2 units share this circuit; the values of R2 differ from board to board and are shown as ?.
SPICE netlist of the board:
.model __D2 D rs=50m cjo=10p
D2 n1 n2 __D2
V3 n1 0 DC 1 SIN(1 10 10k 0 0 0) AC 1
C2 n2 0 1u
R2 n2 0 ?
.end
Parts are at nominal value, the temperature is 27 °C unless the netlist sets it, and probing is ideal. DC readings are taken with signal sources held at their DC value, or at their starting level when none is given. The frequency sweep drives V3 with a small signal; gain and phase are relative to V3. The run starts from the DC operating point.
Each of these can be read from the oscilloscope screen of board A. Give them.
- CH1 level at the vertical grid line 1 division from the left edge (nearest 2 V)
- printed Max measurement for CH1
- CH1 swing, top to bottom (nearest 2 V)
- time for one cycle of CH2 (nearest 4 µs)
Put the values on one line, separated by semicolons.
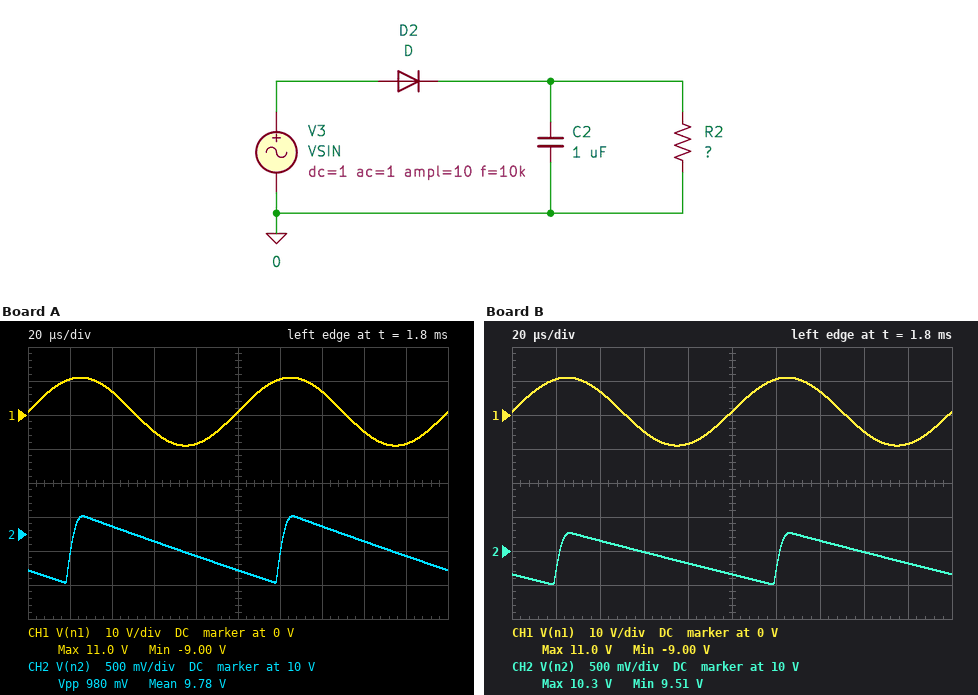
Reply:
10 V; 11.0 V; 20 V; 100 µs
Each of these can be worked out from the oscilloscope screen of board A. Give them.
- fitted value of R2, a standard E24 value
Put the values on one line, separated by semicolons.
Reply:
910 Ω
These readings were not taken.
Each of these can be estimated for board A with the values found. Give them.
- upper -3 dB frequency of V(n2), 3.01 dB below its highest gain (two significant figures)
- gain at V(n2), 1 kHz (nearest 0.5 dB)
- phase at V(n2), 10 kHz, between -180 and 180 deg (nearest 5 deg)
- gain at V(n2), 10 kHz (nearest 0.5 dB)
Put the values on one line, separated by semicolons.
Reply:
2.7 kHz; -1.0 dB; -75 deg; -12.5 dB
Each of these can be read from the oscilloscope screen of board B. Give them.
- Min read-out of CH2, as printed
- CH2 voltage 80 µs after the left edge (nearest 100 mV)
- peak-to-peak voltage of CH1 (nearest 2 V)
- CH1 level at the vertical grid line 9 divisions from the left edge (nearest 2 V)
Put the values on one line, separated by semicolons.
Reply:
9.51 V; 9.8 V; 20 V; -8 V
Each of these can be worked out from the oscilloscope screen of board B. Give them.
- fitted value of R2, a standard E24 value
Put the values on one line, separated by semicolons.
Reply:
1.2 kΩ
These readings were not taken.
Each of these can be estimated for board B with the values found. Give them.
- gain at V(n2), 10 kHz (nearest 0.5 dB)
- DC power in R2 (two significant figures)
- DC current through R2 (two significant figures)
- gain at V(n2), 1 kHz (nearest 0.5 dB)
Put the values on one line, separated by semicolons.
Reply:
-14.5 dB; 120 µW; 310 µA; -1.5 dB
